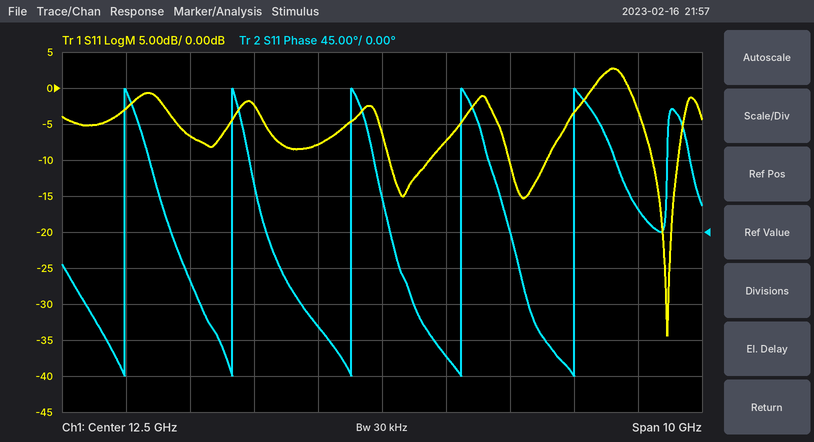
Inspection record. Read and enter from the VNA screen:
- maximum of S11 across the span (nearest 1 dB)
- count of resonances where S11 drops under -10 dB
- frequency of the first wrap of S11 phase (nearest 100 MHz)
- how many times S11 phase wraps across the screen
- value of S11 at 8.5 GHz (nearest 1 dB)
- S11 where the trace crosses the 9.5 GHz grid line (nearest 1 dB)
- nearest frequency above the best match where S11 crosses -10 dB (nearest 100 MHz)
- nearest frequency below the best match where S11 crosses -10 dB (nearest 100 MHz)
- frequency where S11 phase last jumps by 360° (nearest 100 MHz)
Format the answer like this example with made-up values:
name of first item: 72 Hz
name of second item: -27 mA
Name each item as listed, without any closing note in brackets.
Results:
maximum of S11 across the span: 3 dB
count of resonances where S11 drops under -10 dB: 3
frequency of the first wrap of S11 phase: 8.5 GHz
how many times S11 phase wraps across the screen: 5
value of S11 at 8.5 GHz: -3 dB
S11 where the trace crosses the 9.5 GHz grid line: -7 dB
nearest frequency above the best match where S11 crosses -10 dB: 17.1 GHz
nearest frequency below the best match where S11 crosses -10 dB: 16.7 GHz
frequency where S11 phase last jumps by 360°: 15.5 GHz
